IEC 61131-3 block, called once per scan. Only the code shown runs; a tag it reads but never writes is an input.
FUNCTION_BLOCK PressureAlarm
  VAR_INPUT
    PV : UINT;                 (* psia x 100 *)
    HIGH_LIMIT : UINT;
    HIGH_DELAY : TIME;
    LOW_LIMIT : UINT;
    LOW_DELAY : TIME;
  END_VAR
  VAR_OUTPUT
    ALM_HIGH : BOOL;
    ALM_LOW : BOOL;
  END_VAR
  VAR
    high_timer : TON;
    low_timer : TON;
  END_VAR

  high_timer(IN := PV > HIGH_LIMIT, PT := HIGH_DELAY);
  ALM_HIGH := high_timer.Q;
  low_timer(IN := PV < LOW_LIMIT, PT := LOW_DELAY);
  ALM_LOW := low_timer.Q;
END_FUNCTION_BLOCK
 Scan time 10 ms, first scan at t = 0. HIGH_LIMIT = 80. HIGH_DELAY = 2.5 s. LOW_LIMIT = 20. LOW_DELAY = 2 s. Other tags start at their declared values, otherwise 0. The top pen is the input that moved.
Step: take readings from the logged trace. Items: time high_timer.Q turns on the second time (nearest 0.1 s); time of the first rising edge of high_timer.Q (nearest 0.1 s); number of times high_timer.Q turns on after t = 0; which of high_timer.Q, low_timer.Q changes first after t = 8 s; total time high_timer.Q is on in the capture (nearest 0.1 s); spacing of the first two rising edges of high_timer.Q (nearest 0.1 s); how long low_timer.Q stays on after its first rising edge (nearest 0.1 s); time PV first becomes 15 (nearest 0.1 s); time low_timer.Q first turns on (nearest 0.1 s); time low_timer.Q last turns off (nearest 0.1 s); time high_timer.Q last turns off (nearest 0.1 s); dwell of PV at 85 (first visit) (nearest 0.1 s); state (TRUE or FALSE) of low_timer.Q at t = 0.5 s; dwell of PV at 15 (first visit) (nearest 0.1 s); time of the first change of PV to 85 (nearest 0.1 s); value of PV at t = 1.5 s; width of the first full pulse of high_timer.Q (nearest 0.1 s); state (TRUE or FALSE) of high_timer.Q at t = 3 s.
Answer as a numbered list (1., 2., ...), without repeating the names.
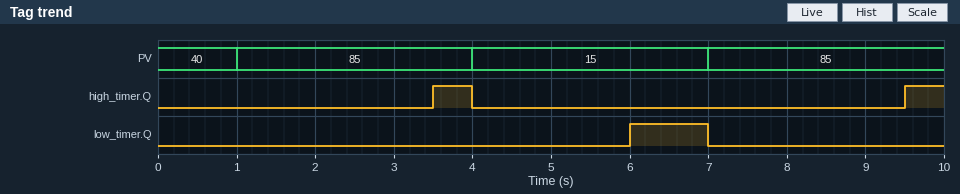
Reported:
1. 9.5 s
2. 3.5 s
3. 2
4. high_timer.Q
5. 1.0 s
6. 6.0 s
7. 1.0 s
8. 4.0 s
9. 6.0 s
10. 7.0 s
11. 4.0 s
12. 3.0 s
13. FALSE
14. 3.0 s
15. 1.0 s
16. 85
17. 0.5 s
18. FALSE
